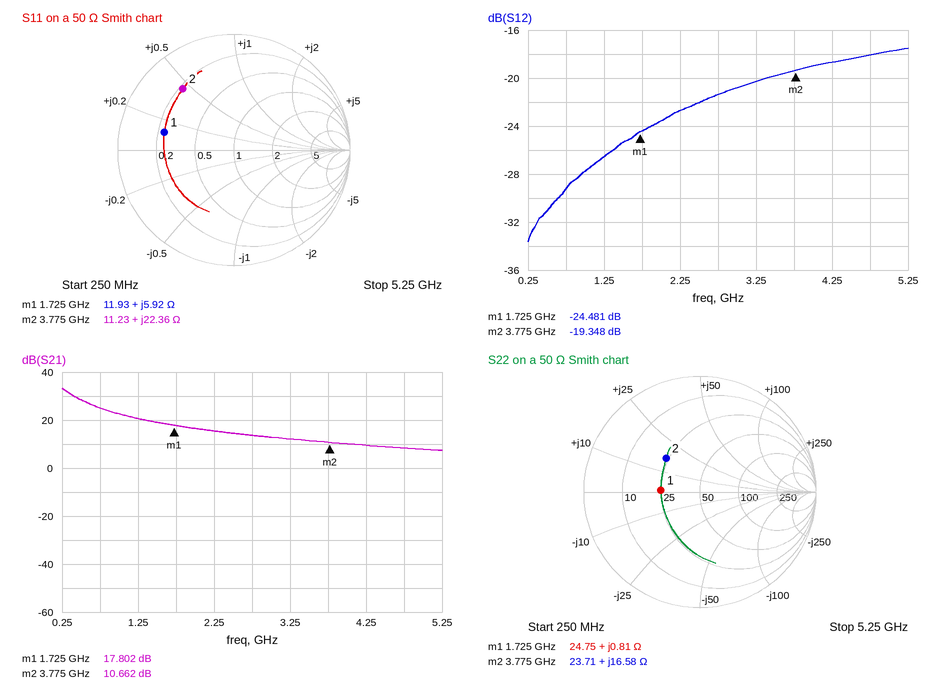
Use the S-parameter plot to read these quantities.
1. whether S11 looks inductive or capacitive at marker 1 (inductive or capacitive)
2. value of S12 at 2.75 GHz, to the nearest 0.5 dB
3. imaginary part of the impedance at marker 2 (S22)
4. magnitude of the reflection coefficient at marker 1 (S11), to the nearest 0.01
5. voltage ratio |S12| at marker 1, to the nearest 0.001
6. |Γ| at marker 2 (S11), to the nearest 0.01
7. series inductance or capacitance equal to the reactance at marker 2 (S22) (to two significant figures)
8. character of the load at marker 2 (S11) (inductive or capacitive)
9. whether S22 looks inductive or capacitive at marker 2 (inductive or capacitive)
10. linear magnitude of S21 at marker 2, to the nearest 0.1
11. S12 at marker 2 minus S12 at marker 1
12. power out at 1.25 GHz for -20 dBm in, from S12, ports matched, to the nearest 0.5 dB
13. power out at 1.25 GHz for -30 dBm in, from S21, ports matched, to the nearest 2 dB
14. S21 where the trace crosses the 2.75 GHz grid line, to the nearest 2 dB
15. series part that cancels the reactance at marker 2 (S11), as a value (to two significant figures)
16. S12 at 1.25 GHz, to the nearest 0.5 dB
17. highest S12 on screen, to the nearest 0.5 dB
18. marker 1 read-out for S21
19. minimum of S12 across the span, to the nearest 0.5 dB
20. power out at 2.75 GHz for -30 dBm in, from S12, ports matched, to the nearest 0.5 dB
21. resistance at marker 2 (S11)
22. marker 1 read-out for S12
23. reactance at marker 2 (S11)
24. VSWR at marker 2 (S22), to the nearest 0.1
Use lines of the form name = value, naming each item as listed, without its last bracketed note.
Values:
whether S11 looks inductive or capacitive at marker 1 = inductive
value of S12 at 2.75 GHz, to the nearest 0.5 dB = -21.5 dB
imaginary part of the impedance at marker 2 = +16.58 Ω
magnitude of the reflection coefficient at marker 1 (S11), to the nearest 0.01 = 0.62
voltage ratio |S12| at marker 1, to the nearest 0.001 = 0.060
|Γ| at marker 2 (S11), to the nearest 0.01 = 0.69
series inductance or capacitance equal to the reactance at marker 2 (S22) = 700 pH
character of the load at marker 2 (S11) = inductive
whether S22 looks inductive or capacitive at marker 2 = inductive
linear magnitude of S21 at marker 2, to the nearest 0.1 = 3.4
S12 at marker 2 minus S12 at marker 1 = 5.133 dB
power out at 1.25 GHz for -20 dBm in, from S12, ports matched, to the nearest 0.5 dB = -46.5 dBm
power out at 1.25 GHz for -30 dBm in, from S21, ports matched, to the nearest 2 dB = -10 dBm
S21 where the trace crosses the 2.75 GHz grid line, to the nearest 2 dB = 14 dB
series part that cancels the reactance at marker 2 (S11), as a value = 1.9 pF
S12 at 1.25 GHz, to the nearest 0.5 dB = -26.5 dB
highest S12 on screen, to the nearest 0.5 dB = -17.5 dB
marker 1 read-out for S21 = 17.802 dB
minimum of S12 across the span, to the nearest 0.5 dB = -33.5 dB
power out at 2.75 GHz for -30 dBm in, from S12, ports matched, to the nearest 0.5 dB = -51.5 dBm
resistance at marker 2 = 11.23 Ω
marker 1 read-out for S12 = -24.481 dB
reactance at marker 2 = +22.36 Ω
VSWR at marker 2 (S22), to the nearest 0.1 = 2.4
